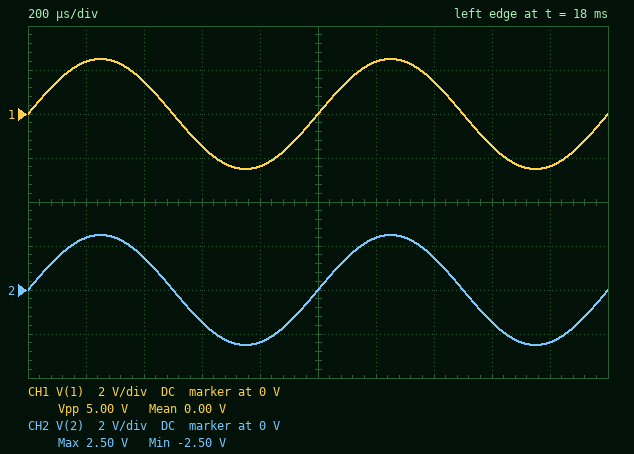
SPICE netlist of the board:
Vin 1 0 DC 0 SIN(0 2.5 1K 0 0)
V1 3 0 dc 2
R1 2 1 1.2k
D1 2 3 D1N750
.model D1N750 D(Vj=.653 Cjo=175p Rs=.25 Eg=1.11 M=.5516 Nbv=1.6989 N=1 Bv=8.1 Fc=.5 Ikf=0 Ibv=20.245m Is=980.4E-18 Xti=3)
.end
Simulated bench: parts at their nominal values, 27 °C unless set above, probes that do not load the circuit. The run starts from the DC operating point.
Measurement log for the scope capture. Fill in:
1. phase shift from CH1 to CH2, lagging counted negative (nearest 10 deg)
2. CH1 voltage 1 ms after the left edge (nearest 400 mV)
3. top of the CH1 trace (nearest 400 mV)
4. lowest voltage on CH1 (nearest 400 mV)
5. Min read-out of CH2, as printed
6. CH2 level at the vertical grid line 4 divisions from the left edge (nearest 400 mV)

0 deg
0 V
2.4 V
-2.4 V
-2.50 V
-2.4 V
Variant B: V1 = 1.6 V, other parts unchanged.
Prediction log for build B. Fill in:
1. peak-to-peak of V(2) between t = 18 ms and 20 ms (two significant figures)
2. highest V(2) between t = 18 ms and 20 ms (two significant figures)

4.8 V
2.3 V
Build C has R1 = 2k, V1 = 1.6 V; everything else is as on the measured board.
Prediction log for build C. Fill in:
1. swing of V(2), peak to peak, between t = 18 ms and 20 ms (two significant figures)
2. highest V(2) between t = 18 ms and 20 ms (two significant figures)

4.8 V
2.3 V
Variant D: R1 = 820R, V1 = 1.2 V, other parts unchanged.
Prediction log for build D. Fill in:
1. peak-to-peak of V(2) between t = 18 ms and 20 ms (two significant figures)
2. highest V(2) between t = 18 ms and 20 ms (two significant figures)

4.4 V
1.9 V
